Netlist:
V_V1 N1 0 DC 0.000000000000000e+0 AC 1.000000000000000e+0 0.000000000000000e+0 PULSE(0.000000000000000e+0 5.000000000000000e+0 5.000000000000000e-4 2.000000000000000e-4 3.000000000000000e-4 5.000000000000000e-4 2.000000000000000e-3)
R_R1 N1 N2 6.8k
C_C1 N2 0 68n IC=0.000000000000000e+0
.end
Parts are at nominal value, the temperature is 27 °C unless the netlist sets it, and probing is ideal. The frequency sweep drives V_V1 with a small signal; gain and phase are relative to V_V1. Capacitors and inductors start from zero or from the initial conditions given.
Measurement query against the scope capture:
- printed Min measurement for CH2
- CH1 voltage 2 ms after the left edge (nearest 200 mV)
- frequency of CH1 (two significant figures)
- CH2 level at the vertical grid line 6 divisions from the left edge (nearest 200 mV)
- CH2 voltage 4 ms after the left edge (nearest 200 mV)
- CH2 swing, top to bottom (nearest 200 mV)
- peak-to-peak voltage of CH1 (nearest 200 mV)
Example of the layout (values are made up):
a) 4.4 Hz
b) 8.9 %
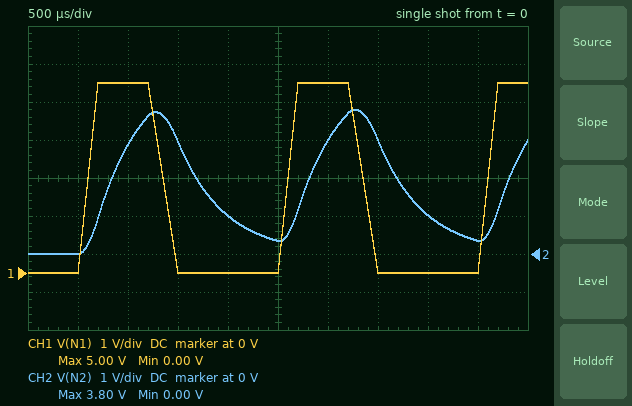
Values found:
a) 0.00 V
b) 0 V
c) 500 Hz
d) 3.0 V
e) 1.0 V
f) 3.8 V
g) 5.0 V
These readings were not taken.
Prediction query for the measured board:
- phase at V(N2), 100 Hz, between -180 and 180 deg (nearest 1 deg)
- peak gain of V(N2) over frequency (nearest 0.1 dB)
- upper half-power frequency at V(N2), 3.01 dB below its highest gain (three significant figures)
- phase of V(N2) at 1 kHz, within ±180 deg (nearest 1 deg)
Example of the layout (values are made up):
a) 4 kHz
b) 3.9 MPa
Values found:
a) -16 deg
b) 0 dB
c) 344 Hz
d) -71 deg
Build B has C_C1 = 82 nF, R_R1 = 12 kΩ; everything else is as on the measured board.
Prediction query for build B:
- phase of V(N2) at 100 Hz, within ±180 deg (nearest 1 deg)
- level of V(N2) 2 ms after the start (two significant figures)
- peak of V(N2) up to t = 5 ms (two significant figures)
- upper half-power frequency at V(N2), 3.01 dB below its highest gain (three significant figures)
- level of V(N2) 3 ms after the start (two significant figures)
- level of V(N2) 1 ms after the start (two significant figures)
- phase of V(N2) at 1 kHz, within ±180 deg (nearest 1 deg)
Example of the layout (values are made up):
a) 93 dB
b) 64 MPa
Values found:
a) -32 deg
b) 1.4 V
c) 2.8 V
d) 162 Hz
e) 2.2 V
f) 1.7 V
g) -81 deg
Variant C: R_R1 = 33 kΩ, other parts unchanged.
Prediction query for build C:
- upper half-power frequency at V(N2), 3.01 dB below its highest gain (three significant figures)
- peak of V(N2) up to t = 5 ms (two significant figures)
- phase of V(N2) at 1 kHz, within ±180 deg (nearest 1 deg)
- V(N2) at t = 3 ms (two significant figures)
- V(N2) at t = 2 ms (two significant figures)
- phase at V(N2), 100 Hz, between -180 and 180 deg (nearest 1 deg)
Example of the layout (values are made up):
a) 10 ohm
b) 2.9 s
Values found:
a) 70.9 Hz
b) 1.9 V
c) -86 deg
d) 1.5 V
e) 1.1 V
f) -55 deg
